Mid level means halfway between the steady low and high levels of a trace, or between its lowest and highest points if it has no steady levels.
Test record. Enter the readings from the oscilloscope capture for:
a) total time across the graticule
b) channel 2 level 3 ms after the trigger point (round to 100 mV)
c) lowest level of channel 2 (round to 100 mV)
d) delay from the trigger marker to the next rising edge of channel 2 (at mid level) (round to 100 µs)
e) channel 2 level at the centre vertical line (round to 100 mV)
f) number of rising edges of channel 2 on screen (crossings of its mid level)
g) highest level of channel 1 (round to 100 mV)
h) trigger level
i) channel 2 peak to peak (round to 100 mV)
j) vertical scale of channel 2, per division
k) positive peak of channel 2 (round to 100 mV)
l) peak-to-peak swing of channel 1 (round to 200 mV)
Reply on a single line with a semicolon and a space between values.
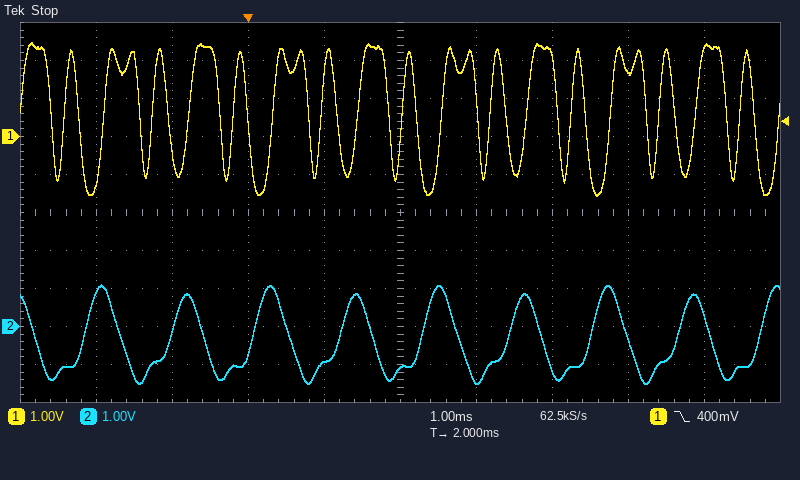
10 ms; -1.4 V; -1.5 V; 100 µs; -1.1 V; 9; 2.5 V; 400 mV; 2.6 V; 1 V; 1.1 V; 4.0 V
